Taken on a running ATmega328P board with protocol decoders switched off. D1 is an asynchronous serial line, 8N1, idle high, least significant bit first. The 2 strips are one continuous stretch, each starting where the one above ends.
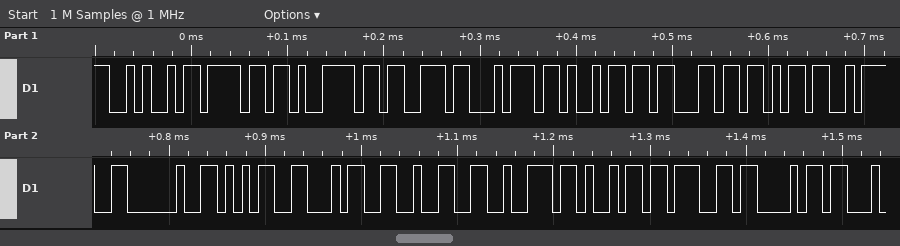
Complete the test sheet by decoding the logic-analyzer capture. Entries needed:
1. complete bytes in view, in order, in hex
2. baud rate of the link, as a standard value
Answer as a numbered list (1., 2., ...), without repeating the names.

1. 4A 6F 79 73 74 69 63 6B 3A 20 35 34 32 72 69 67 68
2. 115200 baud
